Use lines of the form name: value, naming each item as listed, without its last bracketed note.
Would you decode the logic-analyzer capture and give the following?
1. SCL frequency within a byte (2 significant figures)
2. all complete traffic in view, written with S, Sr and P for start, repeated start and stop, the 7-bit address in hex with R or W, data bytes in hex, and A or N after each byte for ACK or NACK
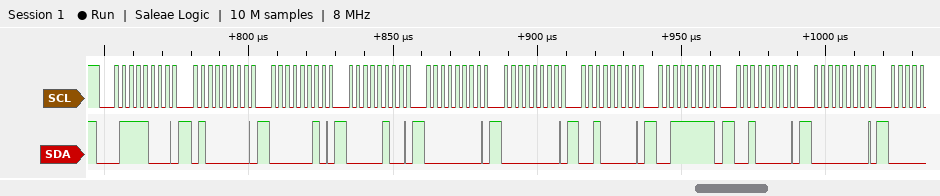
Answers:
SCL frequency within a byte: 400 kHz
all complete traffic in view, written with S, Sr and P for start, repeated start and stop, the 7-bit address in hex with R or W, data bytes in hex, and A or N after each byte for ACK or NACK: S 3CW A 40 A 02 A 04 A 00 A 00 A 20 A 3F A 20 A 00 A
